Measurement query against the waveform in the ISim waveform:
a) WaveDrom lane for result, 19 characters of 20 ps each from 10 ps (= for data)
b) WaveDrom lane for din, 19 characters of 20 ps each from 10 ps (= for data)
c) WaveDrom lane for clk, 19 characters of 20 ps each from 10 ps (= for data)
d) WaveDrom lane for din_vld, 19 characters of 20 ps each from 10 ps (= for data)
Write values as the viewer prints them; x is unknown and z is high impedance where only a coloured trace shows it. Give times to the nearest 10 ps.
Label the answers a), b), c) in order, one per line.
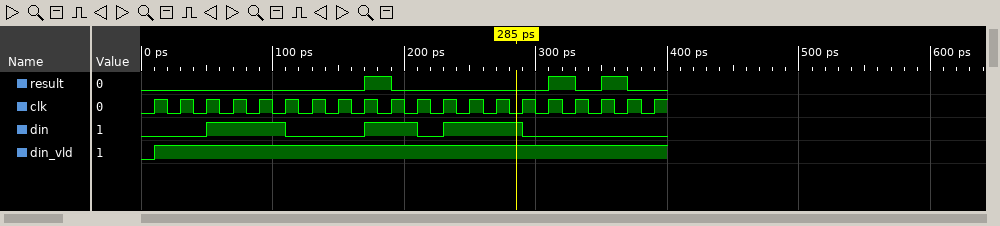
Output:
a) {name: 'result', wave: '0.......10.....1010'}
b) {name: 'din', wave: '0.1..0..1.01..0....'}
c) {name: 'clk', wave: 'p..................'}
d) {name: 'din_vld', wave: '1..................'}
